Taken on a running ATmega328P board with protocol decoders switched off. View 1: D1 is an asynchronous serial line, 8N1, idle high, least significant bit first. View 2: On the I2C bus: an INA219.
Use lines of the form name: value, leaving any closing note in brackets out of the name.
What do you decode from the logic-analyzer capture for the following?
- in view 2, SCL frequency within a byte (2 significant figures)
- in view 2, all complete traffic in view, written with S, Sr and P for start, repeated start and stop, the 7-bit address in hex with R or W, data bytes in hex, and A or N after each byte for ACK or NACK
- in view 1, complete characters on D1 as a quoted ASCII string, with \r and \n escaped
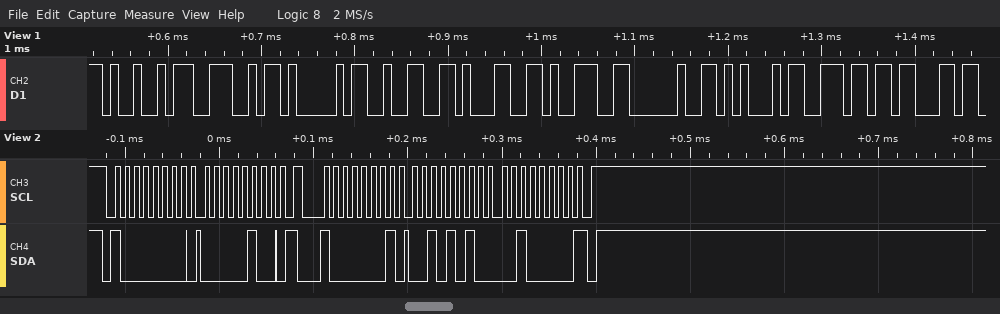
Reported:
in view 2, SCL frequency within a byte: 100 kHz
in view 2, all complete traffic in view, written with S, Sr and P for start, repeated start and stop, the 7-bit address in hex with R or W, data bytes in hex, and A or N after each byte for ACK or NACK: S 40W A 04 A Sr 40R A 2A A 20 N P
in view 1, complete characters on D1 as a quoted ASCII string, with \r and \n escaped: "INA219 Enc"
